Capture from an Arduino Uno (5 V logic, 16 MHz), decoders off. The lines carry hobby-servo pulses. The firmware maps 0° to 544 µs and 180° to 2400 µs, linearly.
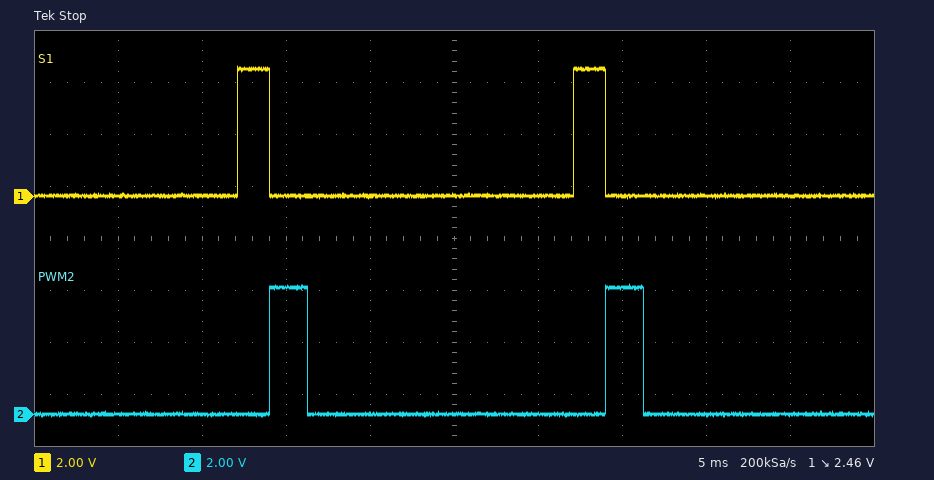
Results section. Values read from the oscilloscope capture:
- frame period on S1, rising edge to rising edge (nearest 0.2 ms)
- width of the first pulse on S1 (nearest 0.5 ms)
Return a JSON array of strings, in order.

["20.0 ms", "2.0 ms"]
